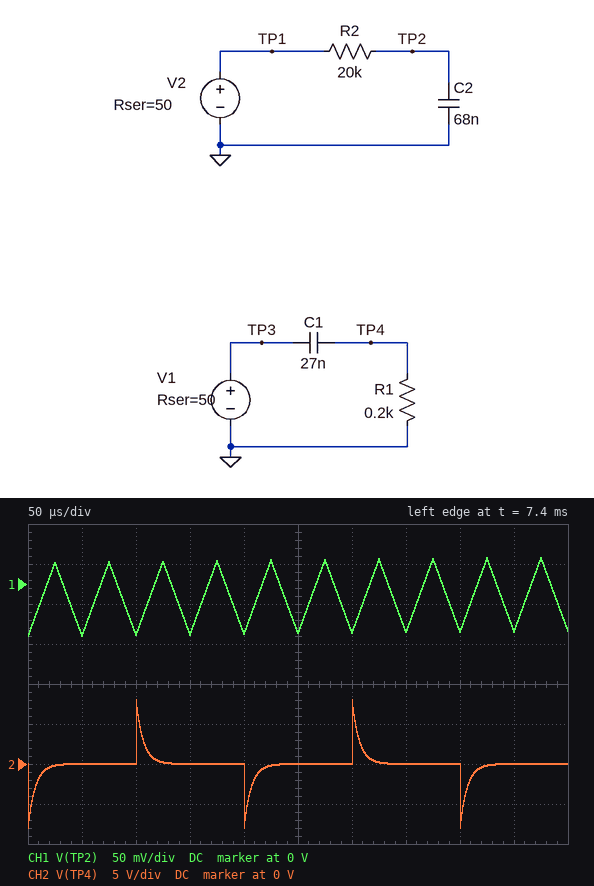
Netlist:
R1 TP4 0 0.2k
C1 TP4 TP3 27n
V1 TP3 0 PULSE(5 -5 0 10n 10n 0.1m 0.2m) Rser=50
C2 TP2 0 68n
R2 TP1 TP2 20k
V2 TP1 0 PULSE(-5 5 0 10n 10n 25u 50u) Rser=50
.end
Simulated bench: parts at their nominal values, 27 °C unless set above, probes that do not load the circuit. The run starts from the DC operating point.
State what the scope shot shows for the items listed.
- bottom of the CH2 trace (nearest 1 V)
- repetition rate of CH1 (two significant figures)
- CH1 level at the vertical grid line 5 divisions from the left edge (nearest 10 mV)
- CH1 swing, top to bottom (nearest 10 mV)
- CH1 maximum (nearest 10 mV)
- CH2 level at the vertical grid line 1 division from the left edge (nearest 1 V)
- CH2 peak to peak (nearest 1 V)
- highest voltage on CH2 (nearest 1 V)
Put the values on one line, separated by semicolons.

-8 V; 20 kHz; -60 mV; 100 mV; 30 mV; 0 V; 16 V; 8 V
